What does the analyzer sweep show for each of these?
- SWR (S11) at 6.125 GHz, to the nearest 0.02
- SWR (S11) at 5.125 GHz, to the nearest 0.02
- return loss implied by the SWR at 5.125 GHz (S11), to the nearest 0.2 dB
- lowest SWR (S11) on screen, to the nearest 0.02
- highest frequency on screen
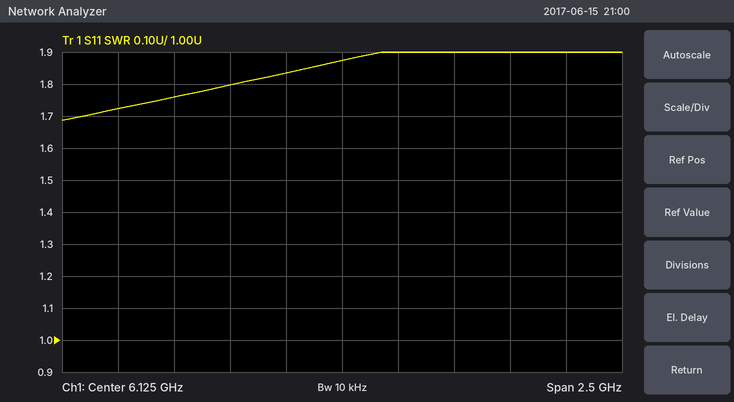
1.88
1.72
11.6 dB
1.68
7.375 GHz
